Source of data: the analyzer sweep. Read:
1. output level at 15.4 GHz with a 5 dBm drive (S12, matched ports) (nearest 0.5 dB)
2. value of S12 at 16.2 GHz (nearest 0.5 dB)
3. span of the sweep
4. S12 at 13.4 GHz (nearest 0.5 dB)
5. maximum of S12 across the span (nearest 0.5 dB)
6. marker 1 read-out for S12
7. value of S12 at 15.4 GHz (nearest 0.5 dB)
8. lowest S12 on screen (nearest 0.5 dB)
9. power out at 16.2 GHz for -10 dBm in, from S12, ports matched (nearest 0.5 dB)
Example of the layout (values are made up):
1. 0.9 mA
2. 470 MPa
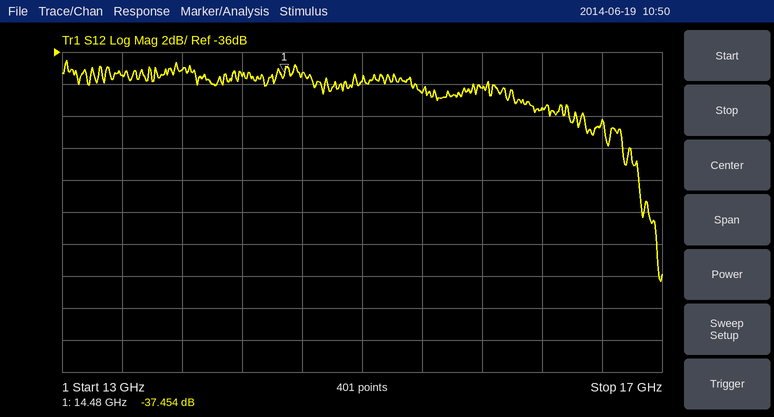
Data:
1. -33.5 dBm
2. -39.5 dB
3. 4 GHz
4. -37.5 dB
5. -36.5 dB
6. -37.454 dB
7. -38.5 dB
8. -50.5 dB
9. -49.5 dBm
